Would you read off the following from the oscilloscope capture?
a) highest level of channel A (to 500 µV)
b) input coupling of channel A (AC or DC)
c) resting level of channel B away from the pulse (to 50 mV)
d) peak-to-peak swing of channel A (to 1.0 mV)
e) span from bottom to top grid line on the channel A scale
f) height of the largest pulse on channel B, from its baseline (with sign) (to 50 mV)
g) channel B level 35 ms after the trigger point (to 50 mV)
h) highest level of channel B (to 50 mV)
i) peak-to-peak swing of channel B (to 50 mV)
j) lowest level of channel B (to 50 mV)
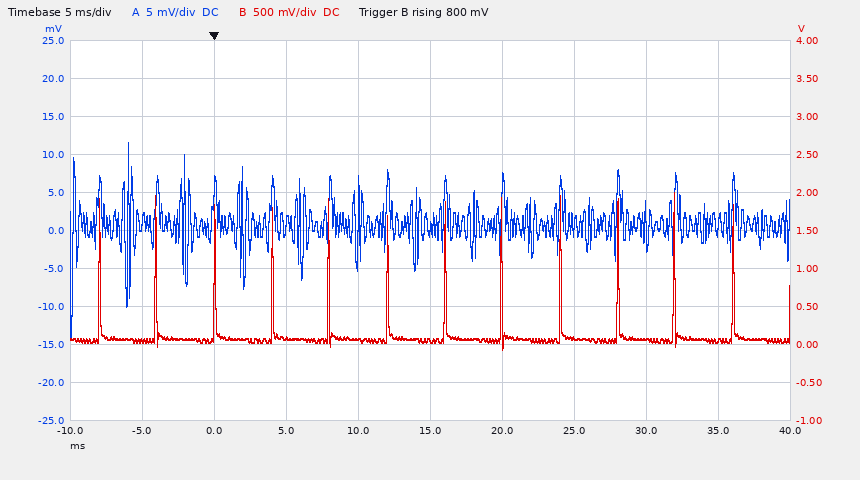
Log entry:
11.5 mV
DC
50 mV
26.0 mV
50 mV
+1.95 V
50 mV
2.00 V
2.05 V
-50 mV
